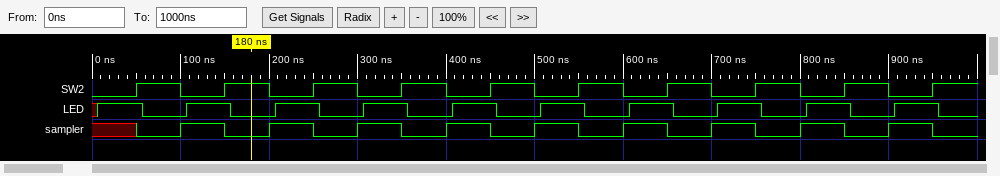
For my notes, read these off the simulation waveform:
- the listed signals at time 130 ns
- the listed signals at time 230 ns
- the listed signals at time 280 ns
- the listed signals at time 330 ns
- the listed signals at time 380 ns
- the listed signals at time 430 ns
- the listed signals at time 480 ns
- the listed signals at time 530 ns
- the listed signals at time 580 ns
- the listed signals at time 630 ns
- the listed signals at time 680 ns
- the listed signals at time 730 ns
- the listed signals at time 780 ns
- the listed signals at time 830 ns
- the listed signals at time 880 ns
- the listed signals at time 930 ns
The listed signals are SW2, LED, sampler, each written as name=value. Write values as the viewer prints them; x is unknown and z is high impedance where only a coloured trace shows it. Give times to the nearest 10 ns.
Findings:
SW2=0, LED=1, sampler=1
SW2=0, LED=1, sampler=1
SW2=1, LED=0, sampler=0
SW2=0, LED=1, sampler=1
SW2=1, LED=0, sampler=0
SW2=0, LED=1, sampler=1
SW2=1, LED=0, sampler=0
SW2=0, LED=1, sampler=1
SW2=1, LED=0, sampler=0
SW2=0, LED=1, sampler=1
SW2=1, LED=0, sampler=0
SW2=0, LED=1, sampler=1
SW2=1, LED=0, sampler=0
SW2=0, LED=1, sampler=1
SW2=1, LED=0, sampler=0
SW2=0, LED=1, sampler=1
